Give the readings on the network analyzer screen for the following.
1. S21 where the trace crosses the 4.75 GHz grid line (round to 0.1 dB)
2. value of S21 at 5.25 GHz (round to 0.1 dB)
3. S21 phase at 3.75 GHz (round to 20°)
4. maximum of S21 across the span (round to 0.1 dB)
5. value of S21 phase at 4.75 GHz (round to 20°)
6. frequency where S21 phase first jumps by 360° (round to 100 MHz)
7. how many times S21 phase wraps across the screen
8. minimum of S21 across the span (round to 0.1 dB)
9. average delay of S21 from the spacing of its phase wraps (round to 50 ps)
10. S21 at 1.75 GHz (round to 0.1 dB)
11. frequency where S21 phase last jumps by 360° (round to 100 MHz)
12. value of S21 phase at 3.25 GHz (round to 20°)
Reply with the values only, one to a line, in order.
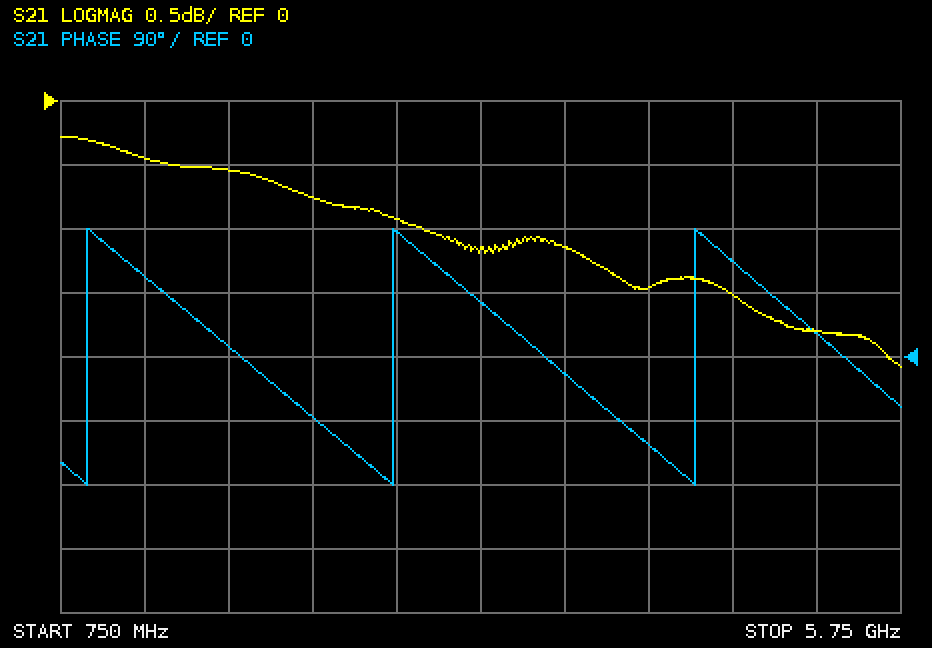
-1.5 dB
-1.8 dB
-20°
-0.3 dB
140°
900 MHz
3
-2.1 dB
550 ps
-0.5 dB
4.5 GHz
80°
